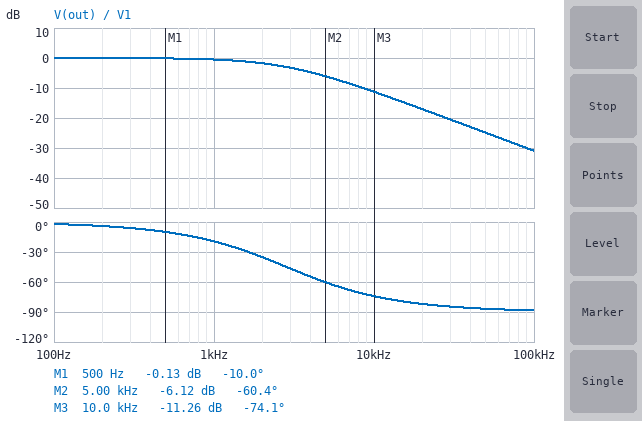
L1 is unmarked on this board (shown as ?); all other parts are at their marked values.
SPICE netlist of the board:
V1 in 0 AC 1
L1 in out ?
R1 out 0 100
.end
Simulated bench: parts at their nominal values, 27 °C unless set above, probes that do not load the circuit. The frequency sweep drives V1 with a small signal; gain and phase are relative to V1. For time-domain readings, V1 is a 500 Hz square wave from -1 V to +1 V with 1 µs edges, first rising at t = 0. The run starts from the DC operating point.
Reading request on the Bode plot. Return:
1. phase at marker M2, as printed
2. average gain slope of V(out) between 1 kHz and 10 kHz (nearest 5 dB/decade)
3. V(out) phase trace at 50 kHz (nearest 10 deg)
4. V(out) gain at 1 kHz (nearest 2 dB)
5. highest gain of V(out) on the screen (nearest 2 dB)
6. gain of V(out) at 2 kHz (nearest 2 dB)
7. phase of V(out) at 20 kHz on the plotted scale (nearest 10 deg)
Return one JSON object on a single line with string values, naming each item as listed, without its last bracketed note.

{"phase at marker M2, as printed": "-60.4 deg", "average gain slope of V(out) between 1 kHz and 10 kHz": "-10 dB/decade", "V(out) phase trace at 50 kHz": "-90 deg", "V(out) gain at 1 kHz": "0 dB", "highest gain of V(out) on the screen": "0 dB", "gain of V(out) at 2 kHz": "-2 dB", "phase of V(out) at 20 kHz on the plotted scale": "-80 deg"}
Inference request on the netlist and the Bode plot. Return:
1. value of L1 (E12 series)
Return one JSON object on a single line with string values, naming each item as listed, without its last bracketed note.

{"value of L1": "5.6 mH"}
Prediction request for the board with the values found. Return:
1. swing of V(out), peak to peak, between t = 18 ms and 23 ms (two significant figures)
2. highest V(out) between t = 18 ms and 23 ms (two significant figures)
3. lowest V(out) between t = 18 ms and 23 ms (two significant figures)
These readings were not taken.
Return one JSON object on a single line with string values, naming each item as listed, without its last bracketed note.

{"swing of V(out), peak to peak, between t = 18 ms and 23 ms": "2.0 V", "highest V(out) between t = 18 ms and 23 ms": "1.0 V", "lowest V(out) between t = 18 ms and 23 ms": "-1.0 V"}
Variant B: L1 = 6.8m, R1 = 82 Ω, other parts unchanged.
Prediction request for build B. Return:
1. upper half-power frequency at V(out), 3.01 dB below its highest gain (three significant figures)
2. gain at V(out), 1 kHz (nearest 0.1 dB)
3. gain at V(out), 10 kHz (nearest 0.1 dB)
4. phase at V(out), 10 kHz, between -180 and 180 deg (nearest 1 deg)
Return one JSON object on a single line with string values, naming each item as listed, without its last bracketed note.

{"upper half-power frequency at V(out), 3.01 dB below its highest gain": "1.92 kHz", "gain at V(out), 1 kHz": "-1.0 dB", "gain at V(out), 10 kHz": "-14.5 dB", "phase at V(out), 10 kHz, between -180 and 180 deg": "-79 deg"}
